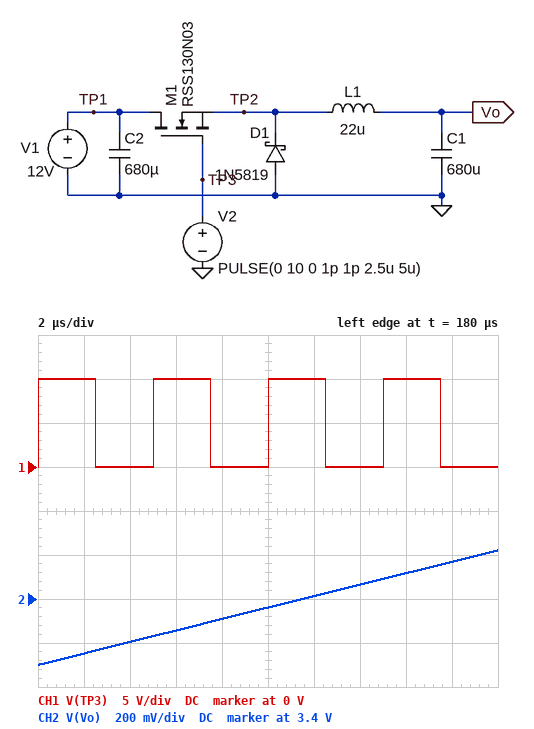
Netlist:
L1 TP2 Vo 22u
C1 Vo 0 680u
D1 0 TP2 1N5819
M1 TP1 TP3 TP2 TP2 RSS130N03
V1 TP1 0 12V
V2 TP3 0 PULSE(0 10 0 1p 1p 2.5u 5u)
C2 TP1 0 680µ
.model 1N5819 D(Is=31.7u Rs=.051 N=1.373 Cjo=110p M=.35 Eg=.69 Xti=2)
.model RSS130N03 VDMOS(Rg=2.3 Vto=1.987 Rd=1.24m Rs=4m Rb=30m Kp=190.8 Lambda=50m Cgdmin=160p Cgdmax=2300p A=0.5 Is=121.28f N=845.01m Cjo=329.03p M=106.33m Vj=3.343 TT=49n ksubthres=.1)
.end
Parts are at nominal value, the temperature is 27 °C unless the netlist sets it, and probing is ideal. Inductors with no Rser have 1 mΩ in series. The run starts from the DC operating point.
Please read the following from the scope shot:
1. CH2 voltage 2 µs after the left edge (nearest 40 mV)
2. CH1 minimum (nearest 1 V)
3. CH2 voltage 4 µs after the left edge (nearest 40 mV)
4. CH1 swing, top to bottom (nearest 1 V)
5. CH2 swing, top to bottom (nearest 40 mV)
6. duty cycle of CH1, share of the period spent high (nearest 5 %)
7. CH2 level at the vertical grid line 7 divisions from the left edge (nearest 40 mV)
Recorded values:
3.16 V
0 V
3.20 V
10 V
520 mV
50 %
3.48 V
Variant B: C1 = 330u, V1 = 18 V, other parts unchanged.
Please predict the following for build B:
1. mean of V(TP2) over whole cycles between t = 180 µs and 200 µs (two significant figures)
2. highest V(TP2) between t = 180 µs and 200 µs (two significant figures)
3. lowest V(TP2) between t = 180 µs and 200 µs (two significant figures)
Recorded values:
3.4 V
7.7 V
-1.0 V
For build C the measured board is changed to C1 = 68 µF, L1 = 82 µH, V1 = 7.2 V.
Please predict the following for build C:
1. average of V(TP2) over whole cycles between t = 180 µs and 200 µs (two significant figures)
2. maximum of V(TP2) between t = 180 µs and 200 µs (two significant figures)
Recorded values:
3.4 V
7.2 V
